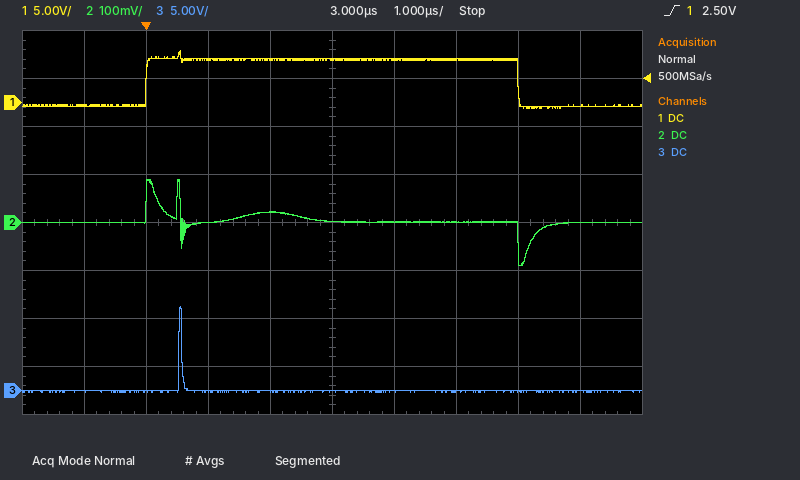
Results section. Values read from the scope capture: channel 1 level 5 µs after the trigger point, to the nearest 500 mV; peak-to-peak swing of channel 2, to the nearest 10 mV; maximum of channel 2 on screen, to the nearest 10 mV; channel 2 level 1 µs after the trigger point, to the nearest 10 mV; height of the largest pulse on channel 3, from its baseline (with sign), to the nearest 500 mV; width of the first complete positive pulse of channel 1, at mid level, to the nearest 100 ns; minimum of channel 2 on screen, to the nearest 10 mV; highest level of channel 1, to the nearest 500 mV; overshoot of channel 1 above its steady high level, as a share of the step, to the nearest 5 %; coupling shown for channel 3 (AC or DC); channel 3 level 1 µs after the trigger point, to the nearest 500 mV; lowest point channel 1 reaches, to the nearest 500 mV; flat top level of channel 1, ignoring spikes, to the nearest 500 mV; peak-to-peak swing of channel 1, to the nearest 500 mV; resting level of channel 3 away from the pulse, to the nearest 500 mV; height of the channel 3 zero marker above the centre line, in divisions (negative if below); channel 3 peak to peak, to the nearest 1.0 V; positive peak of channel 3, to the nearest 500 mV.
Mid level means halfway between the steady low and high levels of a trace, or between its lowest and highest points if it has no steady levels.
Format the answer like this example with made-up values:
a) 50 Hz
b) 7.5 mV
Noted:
a) 4.5 V
b) 180 mV
c) 90 mV
d) 0 mV
e) +9.0 V
f) 6.0 µs
g) -90 mV
h) 5.5 V
i) 20 %
j) DC
k) 0.0 V
l) -500 mV
m) 4.5 V
n) 6.0 V
o) 0.0 V
p) -3.5 div
q) 9.0 V
r) 9.0 V
